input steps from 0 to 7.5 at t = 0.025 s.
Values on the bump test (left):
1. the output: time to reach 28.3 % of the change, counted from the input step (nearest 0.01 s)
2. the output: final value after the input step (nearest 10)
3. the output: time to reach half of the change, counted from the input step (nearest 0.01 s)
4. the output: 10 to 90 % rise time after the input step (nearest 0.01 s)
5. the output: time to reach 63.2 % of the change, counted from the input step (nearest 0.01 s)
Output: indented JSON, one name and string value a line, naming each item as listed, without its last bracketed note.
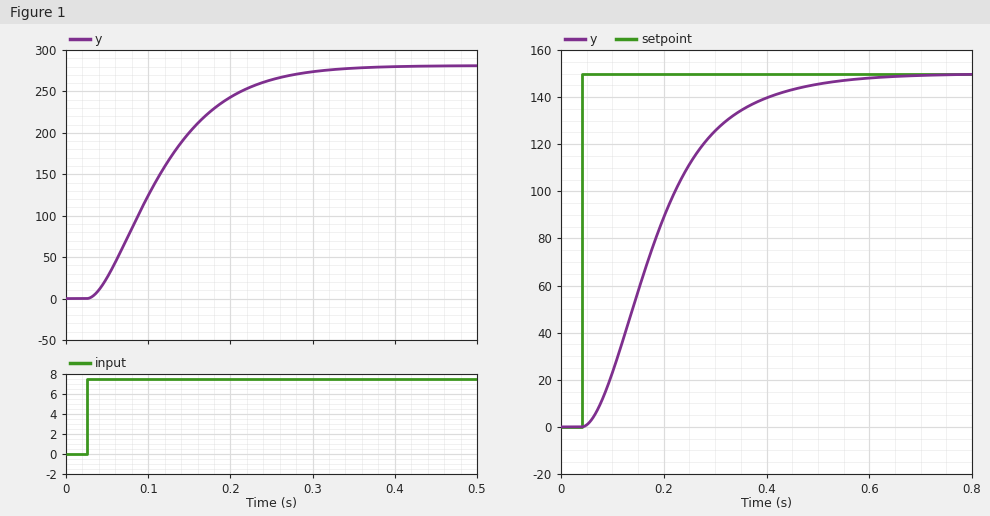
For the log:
{
  "the output: time to reach 28.3 % of the change, counted from the input step": "0.05 s",
  "the output: final value after the input step": "280",
  "the output: time to reach half of the change, counted from the input step": "0.08 s",
  "the output: 10 to 90 % rise time after the input step": "0.17 s",
  "the output: time to reach 63.2 % of the change, counted from the input step": "0.11 s"
}
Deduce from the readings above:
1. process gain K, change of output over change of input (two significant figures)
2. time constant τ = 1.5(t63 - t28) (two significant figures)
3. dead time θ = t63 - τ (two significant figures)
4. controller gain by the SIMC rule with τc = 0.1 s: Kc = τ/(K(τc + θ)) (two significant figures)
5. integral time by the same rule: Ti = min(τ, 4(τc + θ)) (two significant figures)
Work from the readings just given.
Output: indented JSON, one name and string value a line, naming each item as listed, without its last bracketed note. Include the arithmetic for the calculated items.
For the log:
{
  "process gain K, change of output over change of input": "(280 - 0) / 7.5 = 37",
  "time constant τ = 1.5(t63 - t28)": "1.5 × (0.11 - 0.05) = 0.090 s",
  "dead time θ = t63 - τ": "0.11 - 0.09 = 0.020 s",
  "controller gain by the SIMC rule with τc = 0.1 s: Kc = τ/(K(τc + θ))": "0.09 / (37 × (0.1 + 0.02)) = 0.020",
  "integral time by the same rule: Ti = min(τ, 4(τc + θ))": "min(0.09, 4 × (0.1 + 0.02)) = 0.090 s"
}
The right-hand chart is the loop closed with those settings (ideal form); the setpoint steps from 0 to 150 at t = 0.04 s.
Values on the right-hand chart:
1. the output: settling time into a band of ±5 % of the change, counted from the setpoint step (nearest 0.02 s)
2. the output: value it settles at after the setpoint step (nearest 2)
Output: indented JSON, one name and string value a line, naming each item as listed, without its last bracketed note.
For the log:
{
  "the output: settling time into a band of ±5 % of the change, counted from the setpoint step": "0.40 s",
  "the output: value it settles at after the setpoint step": "150"
}
